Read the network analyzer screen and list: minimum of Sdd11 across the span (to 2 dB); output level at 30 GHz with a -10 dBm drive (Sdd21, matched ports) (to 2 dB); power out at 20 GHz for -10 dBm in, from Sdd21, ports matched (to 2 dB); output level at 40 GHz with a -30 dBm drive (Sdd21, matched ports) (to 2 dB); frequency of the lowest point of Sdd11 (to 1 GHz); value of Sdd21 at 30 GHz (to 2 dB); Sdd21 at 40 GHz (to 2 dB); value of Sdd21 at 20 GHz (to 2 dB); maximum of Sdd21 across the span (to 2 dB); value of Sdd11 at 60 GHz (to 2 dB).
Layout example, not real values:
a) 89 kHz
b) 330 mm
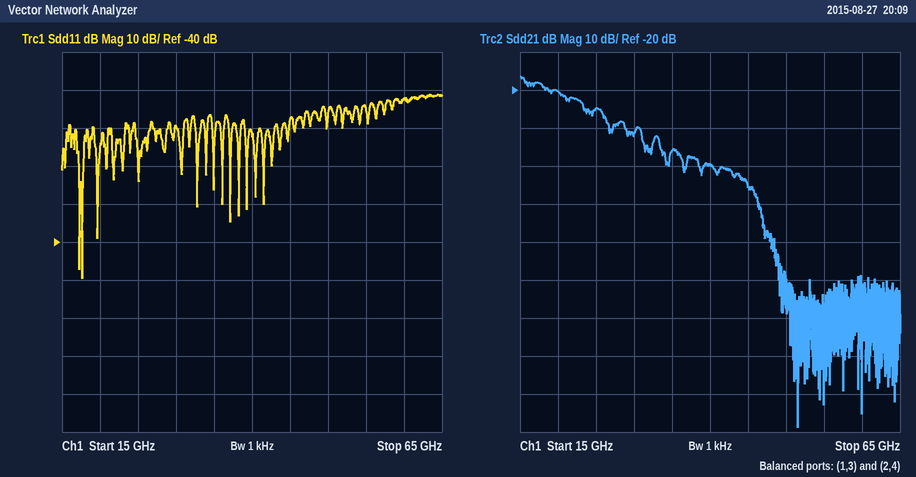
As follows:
a) -50 dB
b) -42 dBm
c) -30 dBm
d) -70 dBm
e) 18 GHz
f) -32 dB
g) -40 dB
h) -20 dB
i) -16 dB
j) -2 dB
